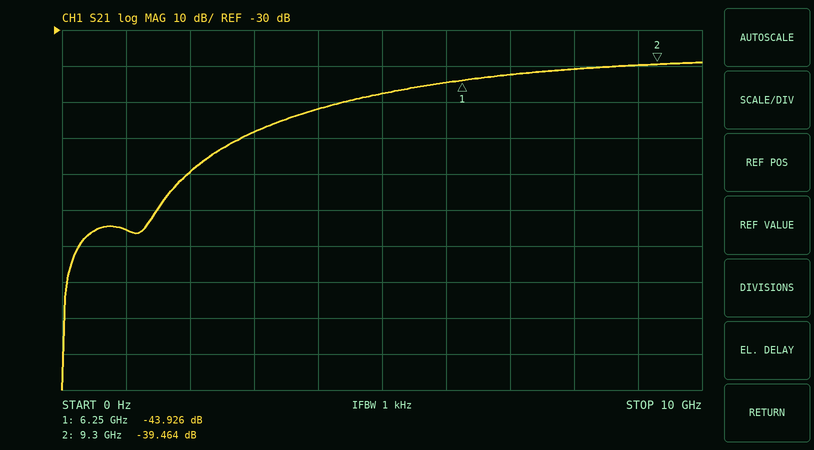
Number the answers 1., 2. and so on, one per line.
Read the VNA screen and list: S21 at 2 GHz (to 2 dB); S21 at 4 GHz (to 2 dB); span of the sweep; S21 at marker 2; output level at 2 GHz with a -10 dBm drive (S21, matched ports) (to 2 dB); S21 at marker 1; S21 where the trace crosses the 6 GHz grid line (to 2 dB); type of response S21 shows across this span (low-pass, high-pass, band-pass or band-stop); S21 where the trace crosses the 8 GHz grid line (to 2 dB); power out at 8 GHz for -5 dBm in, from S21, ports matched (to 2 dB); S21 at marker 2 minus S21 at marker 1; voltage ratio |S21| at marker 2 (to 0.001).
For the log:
1. -70 dB
2. -52 dB
3. 10 GHz
4. -39.464 dB
5. -80 dBm
6. -43.926 dB
7. -44 dB
8. high-pass
9. -40 dB
10. -46 dBm
11. 4.462 dB
12. 0.011
